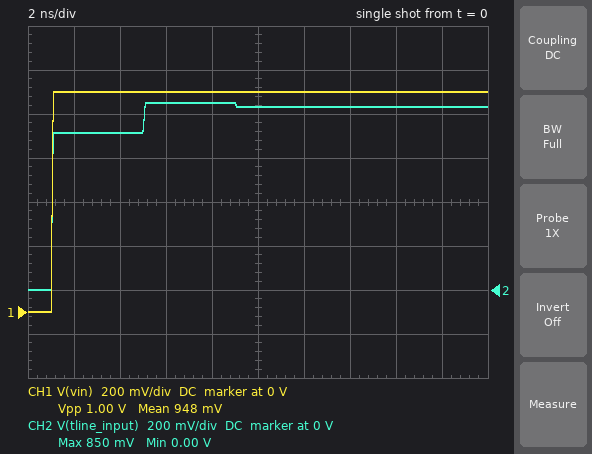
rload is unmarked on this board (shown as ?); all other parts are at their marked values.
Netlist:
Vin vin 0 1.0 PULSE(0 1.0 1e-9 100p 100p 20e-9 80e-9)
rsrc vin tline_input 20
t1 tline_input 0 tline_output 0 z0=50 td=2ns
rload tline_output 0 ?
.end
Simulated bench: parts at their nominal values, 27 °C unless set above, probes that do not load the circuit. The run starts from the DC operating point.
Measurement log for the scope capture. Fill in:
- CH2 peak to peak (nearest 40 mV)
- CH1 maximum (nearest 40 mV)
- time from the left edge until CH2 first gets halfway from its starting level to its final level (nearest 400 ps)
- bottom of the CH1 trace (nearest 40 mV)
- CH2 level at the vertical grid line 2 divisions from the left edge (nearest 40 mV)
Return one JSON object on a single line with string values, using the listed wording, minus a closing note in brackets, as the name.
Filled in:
{"CH2 peak to peak": "840 mV", "CH1 maximum": "1.00 V", "time from the left edge until CH2 first gets halfway from its starting level to its final level": "1.2 ns", "bottom of the CH1 trace": "0 V", "CH2 level at the vertical grid line 2 divisions from the left edge": "720 mV"}
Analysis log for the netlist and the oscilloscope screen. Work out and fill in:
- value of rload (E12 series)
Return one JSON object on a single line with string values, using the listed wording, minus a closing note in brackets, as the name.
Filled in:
{"value of rload": "100 Ω"}
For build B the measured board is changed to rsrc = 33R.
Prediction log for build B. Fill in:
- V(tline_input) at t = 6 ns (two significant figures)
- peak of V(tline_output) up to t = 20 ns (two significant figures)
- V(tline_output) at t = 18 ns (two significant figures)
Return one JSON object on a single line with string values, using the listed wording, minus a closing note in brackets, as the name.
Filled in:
{"V(tline_input) at t = 6 ns": "760 mV", "peak of V(tline_output) up to t = 20 ns": "800 mV", "V(tline_output) at t = 18 ns": "750 mV"}
